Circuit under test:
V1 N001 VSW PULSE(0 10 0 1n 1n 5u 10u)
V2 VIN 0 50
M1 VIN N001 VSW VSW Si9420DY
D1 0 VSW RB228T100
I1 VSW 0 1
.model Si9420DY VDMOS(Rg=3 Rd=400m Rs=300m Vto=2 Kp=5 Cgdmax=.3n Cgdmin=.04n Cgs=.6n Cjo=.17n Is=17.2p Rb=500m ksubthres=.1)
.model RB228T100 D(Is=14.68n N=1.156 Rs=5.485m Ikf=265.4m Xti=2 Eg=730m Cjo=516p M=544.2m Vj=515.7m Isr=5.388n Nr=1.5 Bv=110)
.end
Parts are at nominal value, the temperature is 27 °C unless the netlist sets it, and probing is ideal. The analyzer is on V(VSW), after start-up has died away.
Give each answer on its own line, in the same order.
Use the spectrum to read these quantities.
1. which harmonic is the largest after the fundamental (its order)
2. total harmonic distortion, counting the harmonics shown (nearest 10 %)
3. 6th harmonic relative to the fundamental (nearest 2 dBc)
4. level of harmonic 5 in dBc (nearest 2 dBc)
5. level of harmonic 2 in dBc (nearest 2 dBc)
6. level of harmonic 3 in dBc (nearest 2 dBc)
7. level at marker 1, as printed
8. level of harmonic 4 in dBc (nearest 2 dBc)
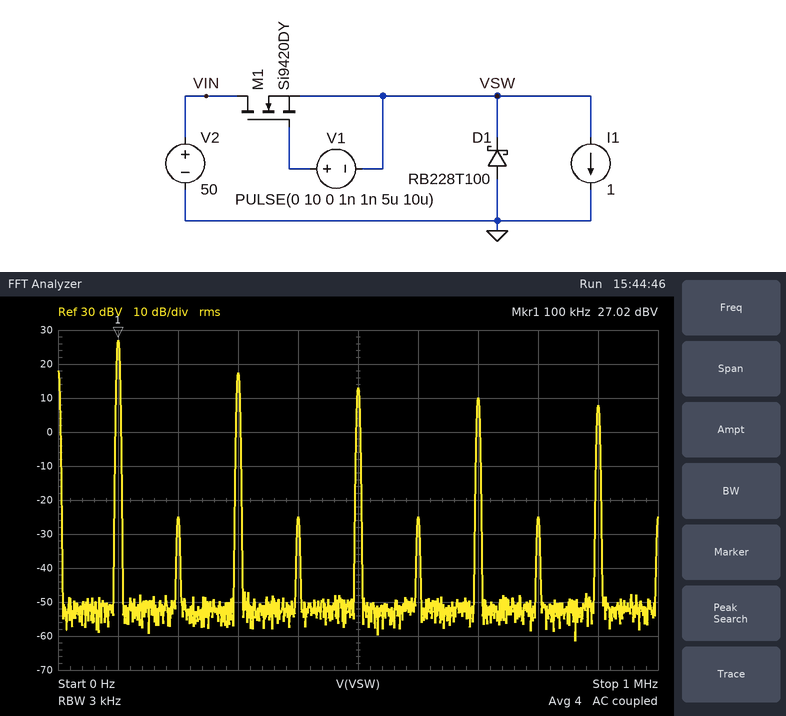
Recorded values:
3
40 %
-52 dBc
-14 dBc
-52 dBc
-10 dBc
27.02 dBV
-52 dBc
